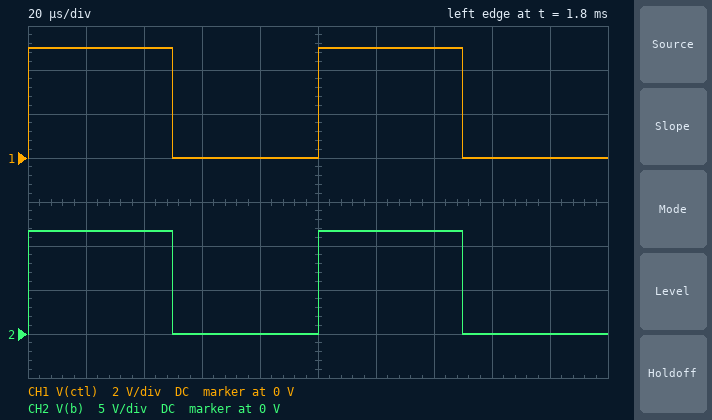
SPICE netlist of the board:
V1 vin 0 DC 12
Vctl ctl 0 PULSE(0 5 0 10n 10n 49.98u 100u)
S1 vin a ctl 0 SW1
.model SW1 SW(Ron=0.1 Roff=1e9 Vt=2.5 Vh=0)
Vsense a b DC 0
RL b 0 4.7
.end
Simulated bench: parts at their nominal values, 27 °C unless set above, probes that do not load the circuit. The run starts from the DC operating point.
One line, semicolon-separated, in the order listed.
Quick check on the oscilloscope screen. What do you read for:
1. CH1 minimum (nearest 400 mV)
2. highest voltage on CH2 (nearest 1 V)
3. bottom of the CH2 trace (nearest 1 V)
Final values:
0 V; 12 V; 0 V
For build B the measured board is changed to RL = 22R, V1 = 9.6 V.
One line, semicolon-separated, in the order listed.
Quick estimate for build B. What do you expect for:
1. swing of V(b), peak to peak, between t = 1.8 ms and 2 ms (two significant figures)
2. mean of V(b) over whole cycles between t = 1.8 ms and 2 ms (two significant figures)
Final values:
9.6 V; 4.8 V
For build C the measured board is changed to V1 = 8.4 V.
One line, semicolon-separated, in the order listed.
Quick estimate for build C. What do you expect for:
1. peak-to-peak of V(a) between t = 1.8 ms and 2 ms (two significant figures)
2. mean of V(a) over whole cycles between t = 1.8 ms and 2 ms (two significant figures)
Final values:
8.2 V; 4.1 V
